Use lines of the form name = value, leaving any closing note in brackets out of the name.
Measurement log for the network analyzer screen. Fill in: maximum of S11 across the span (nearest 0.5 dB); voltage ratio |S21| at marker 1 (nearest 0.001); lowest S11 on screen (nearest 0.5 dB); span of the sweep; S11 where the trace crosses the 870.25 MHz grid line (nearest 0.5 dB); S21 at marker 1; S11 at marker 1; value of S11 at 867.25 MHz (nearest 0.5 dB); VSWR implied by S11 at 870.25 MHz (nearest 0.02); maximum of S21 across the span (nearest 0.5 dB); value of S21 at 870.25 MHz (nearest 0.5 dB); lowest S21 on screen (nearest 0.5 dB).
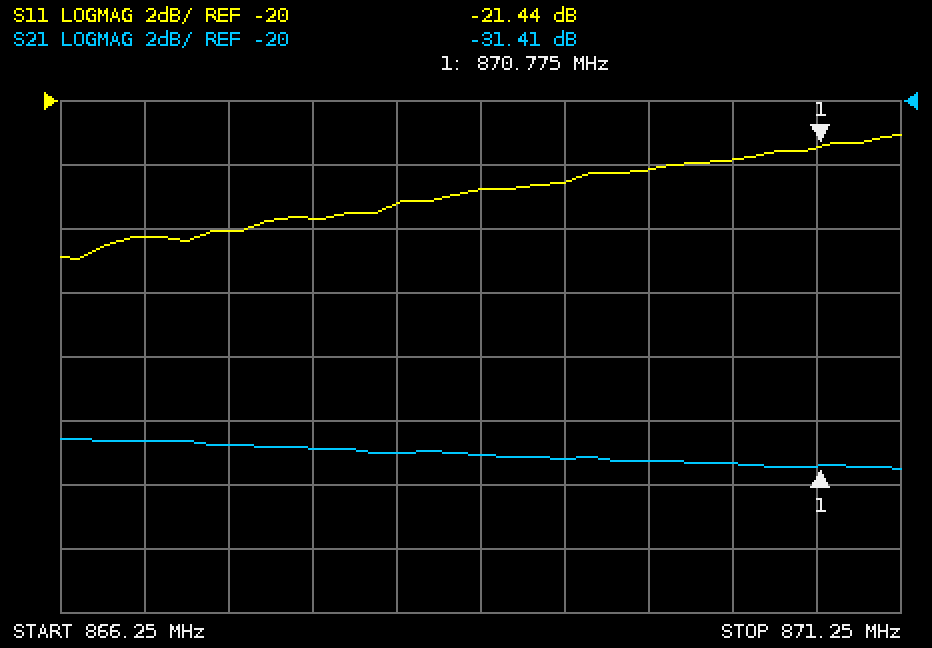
maximum of S11 across the span = -21.0 dB
voltage ratio |S21| at marker 1 = 0.027
lowest S11 on screen = -25.0 dB
span of the sweep = 5 MHz
S11 where the trace crosses the 870.25 MHz grid line = -22.0 dB
S21 at marker 1 = -31.41 dB
S11 at marker 1 = -21.44 dB
value of S11 at 867.25 MHz = -24.0 dB
VSWR implied by S11 at 870.25 MHz = 1.18
maximum of S21 across the span = -30.5 dB
value of S21 at 870.25 MHz = -31.5 dB
lowest S21 on screen = -31.5 dB
